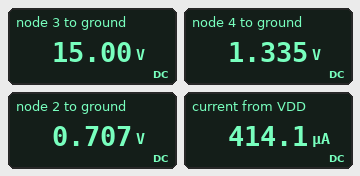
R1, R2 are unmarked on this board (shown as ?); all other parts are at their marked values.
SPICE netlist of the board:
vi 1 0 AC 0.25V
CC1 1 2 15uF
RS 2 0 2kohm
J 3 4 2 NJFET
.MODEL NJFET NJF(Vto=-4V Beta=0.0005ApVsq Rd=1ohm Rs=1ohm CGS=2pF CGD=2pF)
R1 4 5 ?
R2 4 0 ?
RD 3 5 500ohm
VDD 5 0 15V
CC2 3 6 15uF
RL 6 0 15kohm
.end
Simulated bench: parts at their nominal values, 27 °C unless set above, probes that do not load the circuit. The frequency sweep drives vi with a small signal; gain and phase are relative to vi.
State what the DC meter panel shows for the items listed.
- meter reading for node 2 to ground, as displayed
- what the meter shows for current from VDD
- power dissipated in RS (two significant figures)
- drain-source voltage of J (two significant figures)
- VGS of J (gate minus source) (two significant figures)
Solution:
0.707 V
414.1 µA
250 µW
14 V
630 mV
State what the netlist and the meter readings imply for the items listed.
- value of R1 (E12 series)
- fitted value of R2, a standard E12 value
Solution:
33 kΩ
22 kΩ
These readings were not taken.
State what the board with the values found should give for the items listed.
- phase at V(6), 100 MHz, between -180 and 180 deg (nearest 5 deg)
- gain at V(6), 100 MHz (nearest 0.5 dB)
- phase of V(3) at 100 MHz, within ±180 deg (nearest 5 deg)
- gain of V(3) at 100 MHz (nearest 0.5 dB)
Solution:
80 deg
-16.0 dB
80 deg
-16.0 dB
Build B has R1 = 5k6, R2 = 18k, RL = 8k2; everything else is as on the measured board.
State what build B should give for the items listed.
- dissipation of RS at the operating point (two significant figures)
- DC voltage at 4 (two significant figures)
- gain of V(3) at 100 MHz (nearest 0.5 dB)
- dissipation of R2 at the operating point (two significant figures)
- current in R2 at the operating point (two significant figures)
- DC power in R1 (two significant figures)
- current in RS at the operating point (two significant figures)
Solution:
5.9 mW
4.1 V
-15.5 dB
940 µW
230 µA
21 mW
1.7 mA
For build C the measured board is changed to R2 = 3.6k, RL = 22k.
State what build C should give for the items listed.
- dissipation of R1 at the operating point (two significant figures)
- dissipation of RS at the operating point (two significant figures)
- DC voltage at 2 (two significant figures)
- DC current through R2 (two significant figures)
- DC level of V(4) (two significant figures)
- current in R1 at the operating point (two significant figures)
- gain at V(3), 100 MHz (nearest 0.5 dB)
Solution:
6.0 mW
55 µW
330 mV
260 µA
940 mV
430 µA
-16.5 dB
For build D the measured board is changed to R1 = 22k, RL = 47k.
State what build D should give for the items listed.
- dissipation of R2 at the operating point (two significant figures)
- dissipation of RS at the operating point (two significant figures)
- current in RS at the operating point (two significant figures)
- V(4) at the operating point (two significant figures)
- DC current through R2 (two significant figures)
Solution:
130 µW
560 µW
530 µA
1.7 V
77 µA
